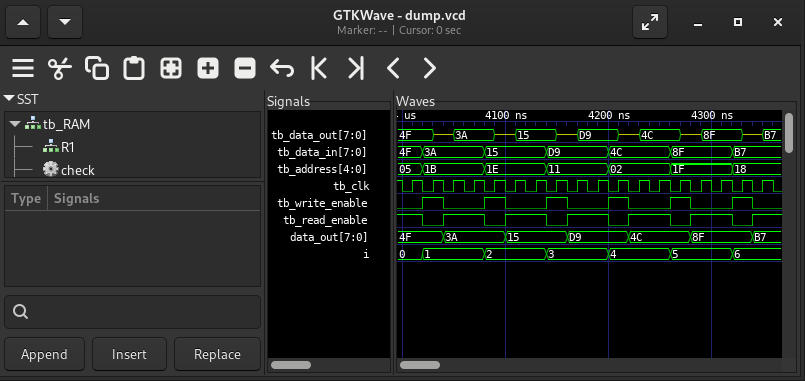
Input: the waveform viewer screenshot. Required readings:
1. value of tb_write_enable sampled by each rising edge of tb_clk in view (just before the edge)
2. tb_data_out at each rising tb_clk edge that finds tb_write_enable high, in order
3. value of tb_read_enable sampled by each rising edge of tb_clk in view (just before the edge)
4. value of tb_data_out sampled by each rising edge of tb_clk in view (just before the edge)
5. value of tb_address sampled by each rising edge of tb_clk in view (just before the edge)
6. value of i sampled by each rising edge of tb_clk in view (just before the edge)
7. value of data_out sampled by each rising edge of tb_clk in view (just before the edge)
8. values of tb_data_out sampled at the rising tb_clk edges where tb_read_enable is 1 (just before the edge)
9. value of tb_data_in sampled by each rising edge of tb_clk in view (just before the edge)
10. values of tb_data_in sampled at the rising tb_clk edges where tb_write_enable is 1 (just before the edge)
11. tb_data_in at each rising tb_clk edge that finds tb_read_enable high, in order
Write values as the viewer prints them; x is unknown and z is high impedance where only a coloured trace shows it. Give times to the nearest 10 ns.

0 1 0 0 1 0 0 1 0 0 1 0 0 1 0 0 1 0
4F, 3A, 15, D9, 4C, 8F
1 0 1 1 0 1 1 0 1 1 0 1 1 0 1 1 0 1
4F, 4F, z, 3A, 3A, z, 15, 15, z, D9, D9, z, 4C, 4C, z, 8F, 8F, z
05, 1B, 1B, 1B, 1E, 1E, 1E, 11, 11, 11, 02, 02, 02, 1F, 1F, 1F, 18, 18
0, 1, 1, 1, 2, 2, 2, 3, 3, 3, 4, 4, 4, 5, 5, 5, 6, 6
4F, 4F, 3A, 3A, 3A, 15, 15, 15, D9, D9, D9, 4C, 4C, 4C, 8F, 8F, 8F, B7
4F, z, 3A, z, 15, z, D9, z, 4C, z, 8F, z
4F, 3A, 3A, 3A, 15, 15, 15, D9, D9, D9, 4C, 4C, 4C, 8F, 8F, 8F, B7, B7
3A, 15, D9, 4C, 8F, B7
4F, 3A, 3A, 15, 15, D9, D9, 4C, 4C, 8F, 8F, B7
